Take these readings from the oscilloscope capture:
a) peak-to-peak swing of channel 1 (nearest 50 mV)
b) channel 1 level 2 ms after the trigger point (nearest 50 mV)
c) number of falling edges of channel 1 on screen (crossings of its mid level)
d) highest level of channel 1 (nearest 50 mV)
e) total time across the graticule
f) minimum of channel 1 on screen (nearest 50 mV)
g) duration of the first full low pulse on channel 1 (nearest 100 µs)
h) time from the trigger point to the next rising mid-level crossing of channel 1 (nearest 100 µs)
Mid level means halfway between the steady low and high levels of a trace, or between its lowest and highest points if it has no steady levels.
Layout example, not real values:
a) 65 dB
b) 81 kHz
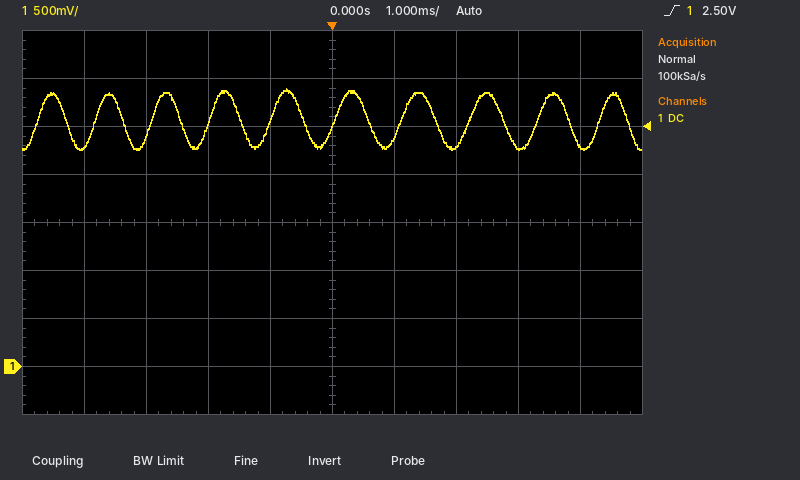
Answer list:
a) 650 mV
b) 2.30 V
c) 10
d) 2.90 V
e) 10 ms
f) 2.25 V
g) 500 µs
h) 1.1 ms
